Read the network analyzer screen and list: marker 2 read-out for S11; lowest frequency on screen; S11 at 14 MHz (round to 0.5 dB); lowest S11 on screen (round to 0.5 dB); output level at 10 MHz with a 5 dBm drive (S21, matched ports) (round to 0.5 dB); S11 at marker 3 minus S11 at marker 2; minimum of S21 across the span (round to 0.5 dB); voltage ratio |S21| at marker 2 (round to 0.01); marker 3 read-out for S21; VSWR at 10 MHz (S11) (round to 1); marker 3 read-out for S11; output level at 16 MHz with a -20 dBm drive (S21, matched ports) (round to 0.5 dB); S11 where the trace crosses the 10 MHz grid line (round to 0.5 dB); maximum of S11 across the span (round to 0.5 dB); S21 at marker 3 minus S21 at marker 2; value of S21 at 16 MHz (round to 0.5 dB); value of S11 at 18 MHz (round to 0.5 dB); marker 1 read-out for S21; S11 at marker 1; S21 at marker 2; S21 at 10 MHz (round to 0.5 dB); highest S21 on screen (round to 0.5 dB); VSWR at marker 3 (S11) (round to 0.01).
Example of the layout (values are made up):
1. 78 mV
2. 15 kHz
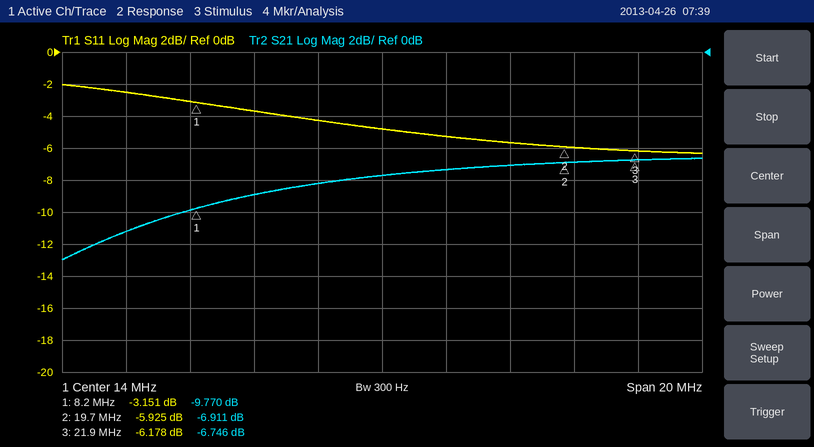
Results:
1. -5.925 dB
2. 4 MHz
3. -5.0 dB
4. -6.5 dB
5. -4.0 dBm
6. -0.253 dB
7. -13.0 dB
8. 0.45
9. -6.746 dB
10. 5
11. -6.178 dB
12. -27.5 dBm
13. -3.5 dB
14. -2.0 dB
15. 0.165 dB
16. -7.5 dB
17. -5.5 dB
18. -9.770 dB
19. -3.151 dB
20. -6.911 dB
21. -9.0 dB
22. -6.5 dB
23. 2.93
